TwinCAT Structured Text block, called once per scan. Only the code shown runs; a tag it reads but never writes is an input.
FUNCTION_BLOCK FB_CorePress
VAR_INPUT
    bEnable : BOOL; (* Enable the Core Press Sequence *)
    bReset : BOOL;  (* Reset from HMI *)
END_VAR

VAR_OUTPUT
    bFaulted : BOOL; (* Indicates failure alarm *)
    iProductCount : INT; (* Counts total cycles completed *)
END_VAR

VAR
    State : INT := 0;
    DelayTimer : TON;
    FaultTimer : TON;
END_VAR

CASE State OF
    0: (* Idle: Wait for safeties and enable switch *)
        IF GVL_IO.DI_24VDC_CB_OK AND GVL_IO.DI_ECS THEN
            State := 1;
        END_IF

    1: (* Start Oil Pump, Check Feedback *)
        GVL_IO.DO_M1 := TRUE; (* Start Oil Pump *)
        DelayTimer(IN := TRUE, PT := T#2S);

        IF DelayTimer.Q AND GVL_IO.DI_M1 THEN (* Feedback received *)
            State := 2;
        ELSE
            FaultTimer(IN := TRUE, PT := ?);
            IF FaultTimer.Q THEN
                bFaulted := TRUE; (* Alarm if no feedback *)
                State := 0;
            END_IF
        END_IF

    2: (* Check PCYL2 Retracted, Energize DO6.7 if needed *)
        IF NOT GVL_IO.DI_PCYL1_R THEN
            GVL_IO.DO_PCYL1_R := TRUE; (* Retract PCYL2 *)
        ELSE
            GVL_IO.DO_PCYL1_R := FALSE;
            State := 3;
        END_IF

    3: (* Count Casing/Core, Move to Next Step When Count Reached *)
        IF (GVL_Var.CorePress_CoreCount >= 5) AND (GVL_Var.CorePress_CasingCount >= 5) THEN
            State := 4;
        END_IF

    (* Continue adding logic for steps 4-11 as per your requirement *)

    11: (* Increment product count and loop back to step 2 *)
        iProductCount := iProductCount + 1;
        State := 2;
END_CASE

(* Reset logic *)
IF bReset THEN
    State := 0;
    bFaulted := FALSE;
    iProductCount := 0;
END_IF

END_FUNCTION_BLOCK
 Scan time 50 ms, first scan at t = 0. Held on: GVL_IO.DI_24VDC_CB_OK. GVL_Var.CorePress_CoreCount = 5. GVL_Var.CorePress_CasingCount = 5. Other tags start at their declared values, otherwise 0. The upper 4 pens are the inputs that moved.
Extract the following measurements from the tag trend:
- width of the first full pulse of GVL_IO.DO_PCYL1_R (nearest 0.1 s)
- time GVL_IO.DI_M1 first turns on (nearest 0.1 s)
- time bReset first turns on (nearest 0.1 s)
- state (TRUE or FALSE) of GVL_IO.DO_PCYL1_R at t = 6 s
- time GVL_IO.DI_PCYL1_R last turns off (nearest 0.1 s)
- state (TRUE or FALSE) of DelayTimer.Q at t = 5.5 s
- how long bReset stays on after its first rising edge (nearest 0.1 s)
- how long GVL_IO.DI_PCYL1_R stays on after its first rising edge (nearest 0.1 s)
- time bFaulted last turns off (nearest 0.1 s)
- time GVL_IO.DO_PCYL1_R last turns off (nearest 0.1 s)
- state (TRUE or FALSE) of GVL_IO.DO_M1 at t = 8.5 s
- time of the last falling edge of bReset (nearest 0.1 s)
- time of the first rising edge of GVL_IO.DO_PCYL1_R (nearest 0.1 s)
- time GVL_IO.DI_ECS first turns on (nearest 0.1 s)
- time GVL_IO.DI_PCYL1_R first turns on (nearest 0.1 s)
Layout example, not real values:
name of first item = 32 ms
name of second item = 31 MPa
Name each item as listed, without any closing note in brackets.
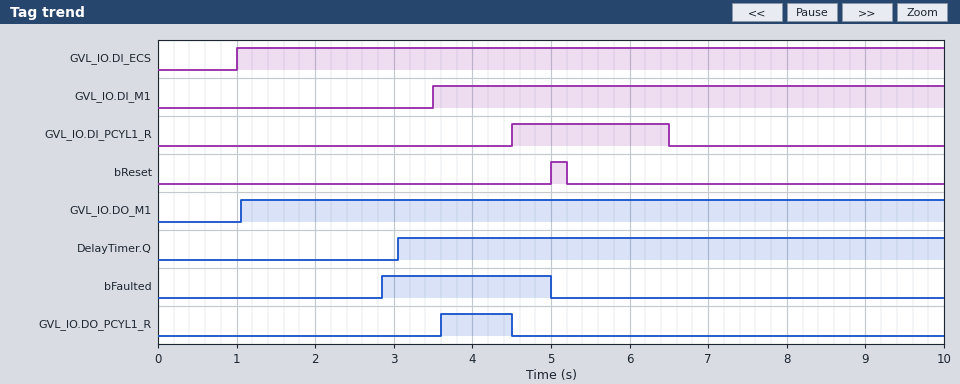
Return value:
width of the first full pulse of GVL_IO.DO_PCYL1_R = 0.9 s
time GVL_IO.DI_M1 first turns on = 3.5 s
time bReset first turns on = 5.0 s
state (TRUE or FALSE) of GVL_IO.DO_PCYL1_R at t = 6 s = FALSE
time GVL_IO.DI_PCYL1_R last turns off = 6.5 s
state (TRUE or FALSE) of DelayTimer.Q at t = 5.5 s = TRUE
how long bReset stays on after its first rising edge = 0.2 s
how long GVL_IO.DI_PCYL1_R stays on after its first rising edge = 2.0 s
time bFaulted last turns off = 5.0 s
time GVL_IO.DO_PCYL1_R last turns off = 4.5 s
state (TRUE or FALSE) of GVL_IO.DO_M1 at t = 8.5 s = TRUE
time of the last falling edge of bReset = 5.2 s
time of the first rising edge of GVL_IO.DO_PCYL1_R = 3.6 s
time GVL_IO.DI_ECS first turns on = 1.0 s
time GVL_IO.DI_PCYL1_R first turns on = 4.5 s
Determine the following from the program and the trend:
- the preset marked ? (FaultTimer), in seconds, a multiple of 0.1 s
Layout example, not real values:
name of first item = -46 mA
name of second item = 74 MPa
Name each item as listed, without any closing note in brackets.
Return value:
the preset marked ? (FaultTimer), in seconds, a multiple of 0.1 s = 1.8 s
